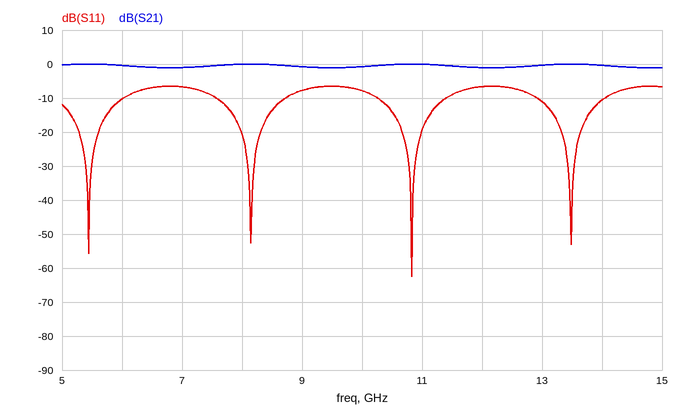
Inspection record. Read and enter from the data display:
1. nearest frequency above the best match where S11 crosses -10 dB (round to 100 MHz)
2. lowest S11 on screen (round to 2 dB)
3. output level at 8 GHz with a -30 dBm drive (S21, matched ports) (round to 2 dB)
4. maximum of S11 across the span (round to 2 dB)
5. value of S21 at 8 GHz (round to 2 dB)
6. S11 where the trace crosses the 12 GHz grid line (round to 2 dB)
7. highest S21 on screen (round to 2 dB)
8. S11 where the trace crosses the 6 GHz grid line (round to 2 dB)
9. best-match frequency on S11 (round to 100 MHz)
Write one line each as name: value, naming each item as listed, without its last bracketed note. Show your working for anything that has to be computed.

nearest frequency above the best match where S11 crosses -10 dB: 11.4 GHz
lowest S11 on screen: -62 dB
output level at 8 GHz with a -30 dBm drive (S21, matched ports): -30 dBm + (0 dB) = -30 dBm
maximum of S11 across the span: -6 dB
value of S21 at 8 GHz: 0 dB
S11 where the trace crosses the 12 GHz grid line: -6 dB
highest S21 on screen: 0 dB
S11 where the trace crosses the 6 GHz grid line: -10 dB
best-match frequency on S11: 10.8 GHz
